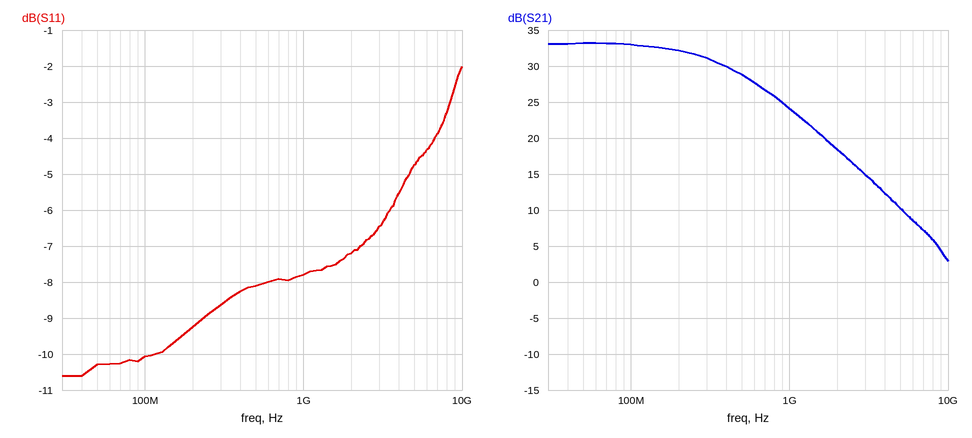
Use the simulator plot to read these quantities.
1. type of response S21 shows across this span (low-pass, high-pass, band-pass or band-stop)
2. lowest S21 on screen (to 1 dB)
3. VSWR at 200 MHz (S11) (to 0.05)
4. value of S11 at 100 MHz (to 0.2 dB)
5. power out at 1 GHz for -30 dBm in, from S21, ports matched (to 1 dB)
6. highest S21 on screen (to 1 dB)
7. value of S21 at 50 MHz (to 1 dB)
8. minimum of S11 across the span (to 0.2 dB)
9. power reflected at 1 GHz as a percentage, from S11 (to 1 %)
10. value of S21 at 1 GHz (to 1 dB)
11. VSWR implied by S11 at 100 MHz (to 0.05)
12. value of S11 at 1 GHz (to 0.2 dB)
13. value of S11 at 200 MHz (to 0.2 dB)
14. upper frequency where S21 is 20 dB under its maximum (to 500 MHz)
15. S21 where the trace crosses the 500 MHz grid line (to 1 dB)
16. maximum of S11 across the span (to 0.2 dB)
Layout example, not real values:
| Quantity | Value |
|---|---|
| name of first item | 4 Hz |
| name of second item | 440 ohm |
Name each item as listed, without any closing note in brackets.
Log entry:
| Quantity | Value |
|---|---|
| type of response S21 shows across this span | low-pass |
| lowest S21 on screen | 3 dB |
| VSWR at 200 MHz (S11) | 2.05 |
| value of S11 at 100 MHz | -10.0 dB |
| power out at 1 GHz for -30 dBm in, from S21, ports matched | -6 dBm |
| highest S21 on screen | 33 dB |
| value of S21 at 50 MHz | 33 dB |
| minimum of S11 across the span | -10.6 dB |
| power reflected at 1 GHz as a percentage, from S11 | 17 % |
| value of S21 at 1 GHz | 24 dB |
| VSWR implied by S11 at 100 MHz | 1.90 |
| value of S11 at 1 GHz | -7.8 dB |
| value of S11 at 200 MHz | -9.2 dB |
| upper frequency where S21 is 20 dB under its maximum | 3.5 GHz |
| S21 where the trace crosses the 500 MHz grid line | 29 dB |
| maximum of S11 across the span | -2.0 dB |
